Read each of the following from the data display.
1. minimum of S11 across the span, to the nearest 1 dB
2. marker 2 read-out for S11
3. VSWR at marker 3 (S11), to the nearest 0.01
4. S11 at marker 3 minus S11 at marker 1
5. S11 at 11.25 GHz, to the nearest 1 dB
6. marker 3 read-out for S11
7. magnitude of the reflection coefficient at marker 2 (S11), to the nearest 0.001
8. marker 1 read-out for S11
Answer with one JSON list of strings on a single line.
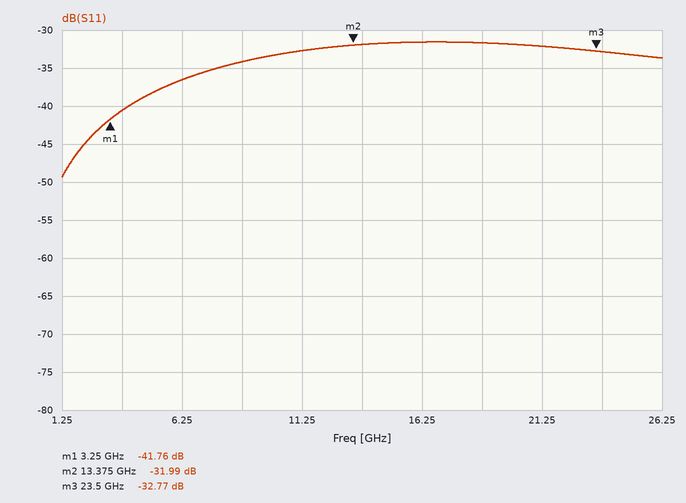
["-49 dB", "-31.99 dB", "1.05", "8.99 dB", "-33 dB", "-32.77 dB", "0.025", "-41.76 dB"]
